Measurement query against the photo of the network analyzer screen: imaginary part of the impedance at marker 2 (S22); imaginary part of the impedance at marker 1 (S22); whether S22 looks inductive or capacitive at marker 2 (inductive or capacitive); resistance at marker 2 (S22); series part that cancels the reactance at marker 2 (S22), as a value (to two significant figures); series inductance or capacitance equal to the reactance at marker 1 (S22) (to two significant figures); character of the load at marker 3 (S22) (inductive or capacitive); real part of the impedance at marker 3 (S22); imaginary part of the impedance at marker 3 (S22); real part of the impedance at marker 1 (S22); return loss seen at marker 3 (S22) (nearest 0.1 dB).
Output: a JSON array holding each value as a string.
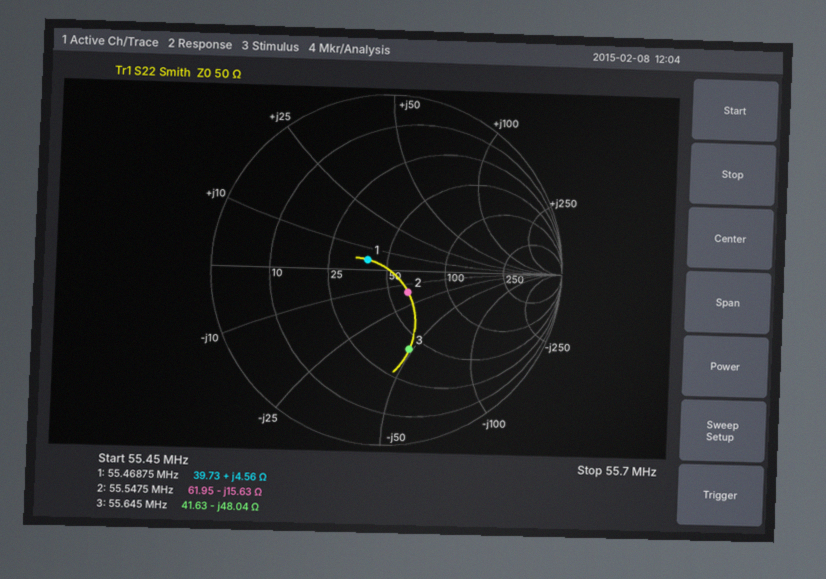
["-15.63 Ω", "+4.56 Ω", "capacitive", "61.95 Ω", "45 nH", "13 nH", "capacitive", "41.63 Ω", "-48.04 Ω", "39.73 Ω", "6.5 dB"]
